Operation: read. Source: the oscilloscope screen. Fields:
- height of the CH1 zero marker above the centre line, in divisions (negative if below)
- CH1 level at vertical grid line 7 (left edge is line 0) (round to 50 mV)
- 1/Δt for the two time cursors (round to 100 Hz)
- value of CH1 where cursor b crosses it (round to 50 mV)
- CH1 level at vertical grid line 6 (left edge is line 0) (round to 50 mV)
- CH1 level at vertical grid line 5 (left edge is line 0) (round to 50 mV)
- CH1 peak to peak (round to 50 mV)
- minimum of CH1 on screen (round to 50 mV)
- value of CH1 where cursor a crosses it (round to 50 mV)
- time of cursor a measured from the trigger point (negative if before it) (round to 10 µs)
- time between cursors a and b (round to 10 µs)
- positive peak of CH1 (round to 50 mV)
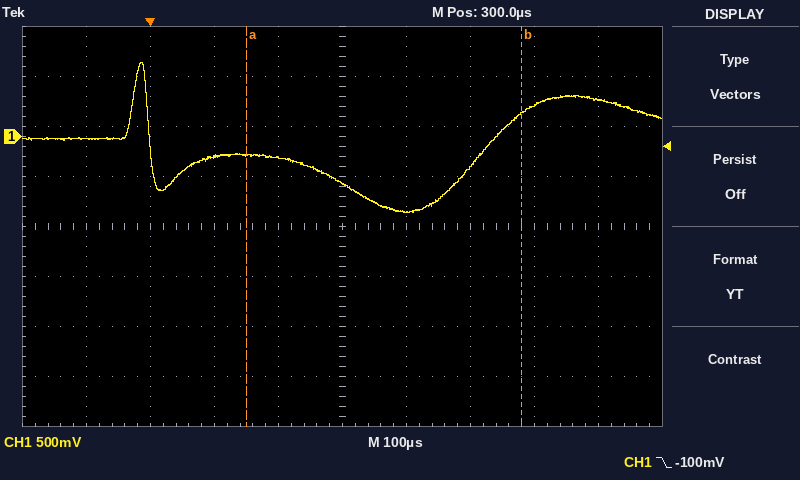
+1.8 div
-300 mV
2.3 kHz
250 mV
-750 mV
-450 mV
1.50 V
-750 mV
-200 mV
+150 µs
430 µs
750 mV
